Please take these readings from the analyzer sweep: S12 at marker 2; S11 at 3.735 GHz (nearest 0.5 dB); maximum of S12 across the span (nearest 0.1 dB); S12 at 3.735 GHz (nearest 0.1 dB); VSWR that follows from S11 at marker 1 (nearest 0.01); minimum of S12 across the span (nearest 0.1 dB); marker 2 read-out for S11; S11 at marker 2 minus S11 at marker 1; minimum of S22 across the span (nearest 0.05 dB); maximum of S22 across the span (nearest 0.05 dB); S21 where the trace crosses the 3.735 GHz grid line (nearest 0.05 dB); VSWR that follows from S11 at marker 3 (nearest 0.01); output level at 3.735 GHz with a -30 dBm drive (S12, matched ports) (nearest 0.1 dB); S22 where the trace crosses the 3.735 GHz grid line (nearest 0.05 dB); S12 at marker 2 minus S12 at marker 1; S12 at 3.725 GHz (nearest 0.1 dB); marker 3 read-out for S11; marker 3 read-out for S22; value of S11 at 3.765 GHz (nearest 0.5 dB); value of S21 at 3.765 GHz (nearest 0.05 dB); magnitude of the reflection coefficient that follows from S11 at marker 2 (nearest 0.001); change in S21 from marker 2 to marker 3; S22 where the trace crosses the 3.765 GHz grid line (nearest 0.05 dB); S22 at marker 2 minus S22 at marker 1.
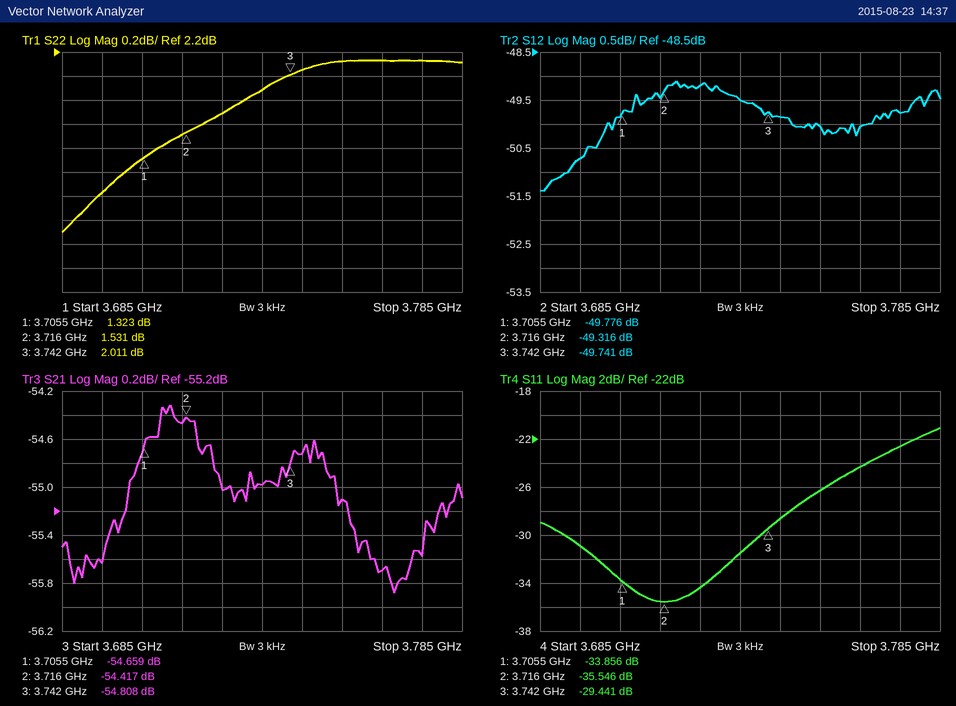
-49.316 dB
-31.5 dB
-49.1 dB
-49.5 dB
1.04
-51.4 dB
-35.546 dB
-1.690 dB
0.70 dB
2.15 dB
-55.00 dB
1.07
-79.5 dBm
1.90 dB
0.460 dB
-49.2 dB
-29.441 dB
2.011 dB
-24.5 dB
-55.70 dB
0.017
-0.391 dB
2.15 dB
0.208 dB
